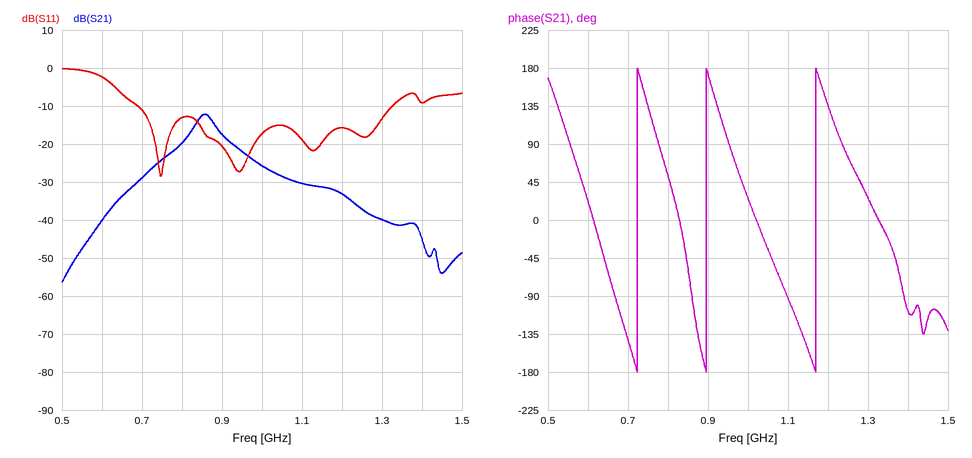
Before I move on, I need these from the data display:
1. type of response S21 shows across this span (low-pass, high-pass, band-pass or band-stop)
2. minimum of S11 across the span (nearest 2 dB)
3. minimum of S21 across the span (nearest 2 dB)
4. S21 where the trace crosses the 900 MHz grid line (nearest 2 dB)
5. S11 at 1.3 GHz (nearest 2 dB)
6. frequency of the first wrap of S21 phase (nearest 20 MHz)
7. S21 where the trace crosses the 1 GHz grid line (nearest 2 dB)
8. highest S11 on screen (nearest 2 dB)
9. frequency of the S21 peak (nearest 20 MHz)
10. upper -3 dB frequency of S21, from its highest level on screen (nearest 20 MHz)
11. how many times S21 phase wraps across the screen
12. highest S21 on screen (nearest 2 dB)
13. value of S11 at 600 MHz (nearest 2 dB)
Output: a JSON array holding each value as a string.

["band-pass", "-28 dB", "-56 dB", "-18 dB", "-14 dB", "720 MHz", "-26 dB", "0 dB", "860 MHz", "880 MHz", "3", "-12 dB", "-2 dB"]
